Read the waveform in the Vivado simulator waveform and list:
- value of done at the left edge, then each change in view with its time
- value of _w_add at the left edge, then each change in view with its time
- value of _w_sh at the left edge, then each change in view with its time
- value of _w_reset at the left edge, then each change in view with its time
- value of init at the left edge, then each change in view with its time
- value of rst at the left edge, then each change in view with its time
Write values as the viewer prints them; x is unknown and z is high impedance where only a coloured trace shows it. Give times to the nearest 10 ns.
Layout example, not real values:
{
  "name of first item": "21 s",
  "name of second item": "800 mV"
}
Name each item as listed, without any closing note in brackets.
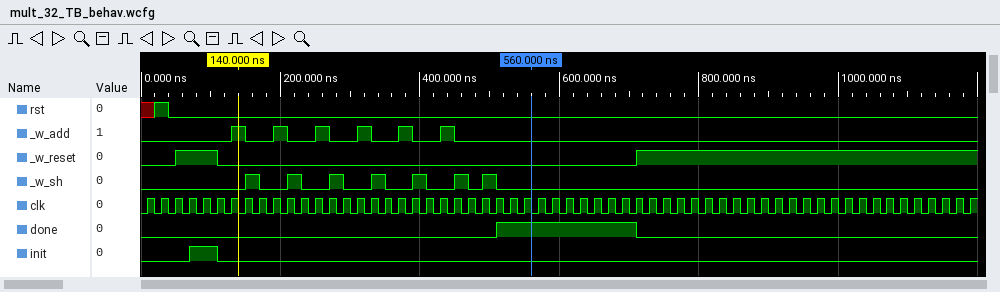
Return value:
{
  "value of done at the left edge, then each change in view with its time": "0, 1 at 510 ns, 0 at 710 ns",
  "value of _w_add at the left edge, then each change in view with its time": "0, 1 at 130 ns, 0 at 150 ns, 1 at 190 ns, 0 at 210 ns, 1 at 250 ns, 0 at 270 ns, 1 at 310 ns, 0 at 330 ns, 1 at 370 ns, 0 at 390 ns, 1 at 430 ns, 0 at 450 ns",
  "value of _w_sh at the left edge, then each change in view with its time": "0, 1 at 150 ns, 0 at 170 ns, 1 at 210 ns, 0 at 230 ns, 1 at 270 ns, 0 at 290 ns, 1 at 330 ns, 0 at 350 ns, 1 at 390 ns, 0 at 410 ns, 1 at 450 ns, 0 at 470 ns, 1 at 490 ns, 0 at 510 ns",
  "value of _w_reset at the left edge, then each change in view with its time": "0, 1 at 50 ns, 0 at 110 ns, 1 at 710 ns",
  "value of init at the left edge, then each change in view with its time": "0, 1 at 70 ns, 0 at 110 ns",
  "value of rst at the left edge, then each change in view with its time": "x, 1 at 20 ns, 0 at 40 ns"
}
